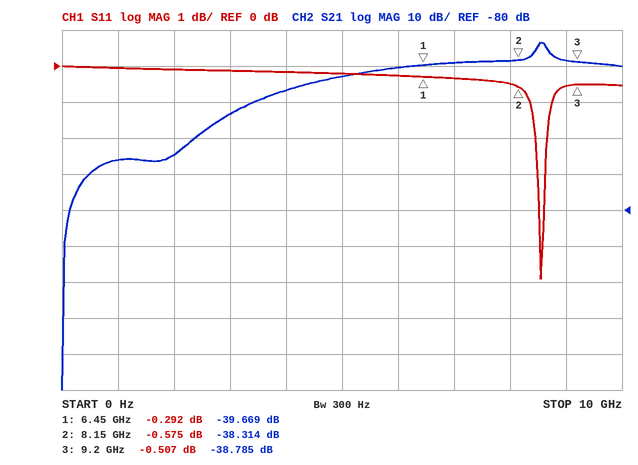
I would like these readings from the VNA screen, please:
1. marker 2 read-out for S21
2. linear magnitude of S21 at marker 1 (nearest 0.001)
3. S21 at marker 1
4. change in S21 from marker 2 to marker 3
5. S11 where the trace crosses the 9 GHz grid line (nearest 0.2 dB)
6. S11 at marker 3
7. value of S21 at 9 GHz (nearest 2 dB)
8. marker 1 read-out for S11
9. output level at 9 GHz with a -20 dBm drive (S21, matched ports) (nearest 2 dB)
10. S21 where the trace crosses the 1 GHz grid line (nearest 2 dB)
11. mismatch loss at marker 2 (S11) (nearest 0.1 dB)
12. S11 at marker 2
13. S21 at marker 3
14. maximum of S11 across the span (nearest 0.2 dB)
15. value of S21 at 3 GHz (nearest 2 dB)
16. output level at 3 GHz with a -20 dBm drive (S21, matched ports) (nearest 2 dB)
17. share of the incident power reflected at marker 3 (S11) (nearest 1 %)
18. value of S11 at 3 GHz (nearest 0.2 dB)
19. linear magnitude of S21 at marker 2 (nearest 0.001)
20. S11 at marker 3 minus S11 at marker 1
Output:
-38.314 dB
0.010
-39.669 dB
-0.471 dB
-0.6 dB
-0.507 dB
-38 dB
-0.292 dB
-58 dBm
-66 dB
9.1 dB
-0.575 dB
-38.785 dB
0.0 dB
-54 dB
-74 dBm
89 %
-0.2 dB
0.012
-0.215 dB
